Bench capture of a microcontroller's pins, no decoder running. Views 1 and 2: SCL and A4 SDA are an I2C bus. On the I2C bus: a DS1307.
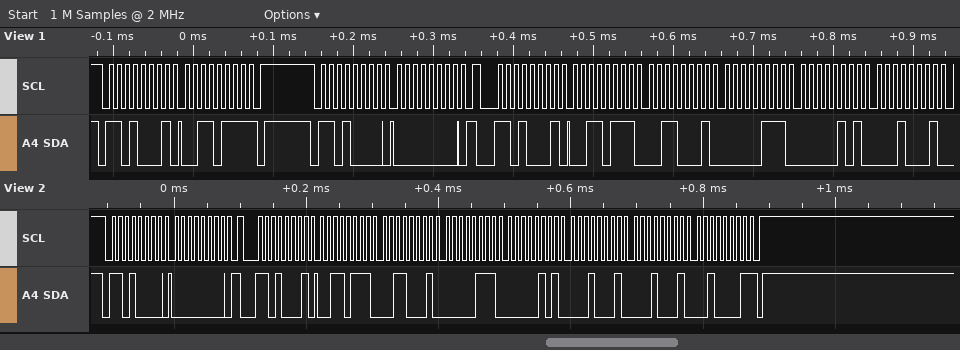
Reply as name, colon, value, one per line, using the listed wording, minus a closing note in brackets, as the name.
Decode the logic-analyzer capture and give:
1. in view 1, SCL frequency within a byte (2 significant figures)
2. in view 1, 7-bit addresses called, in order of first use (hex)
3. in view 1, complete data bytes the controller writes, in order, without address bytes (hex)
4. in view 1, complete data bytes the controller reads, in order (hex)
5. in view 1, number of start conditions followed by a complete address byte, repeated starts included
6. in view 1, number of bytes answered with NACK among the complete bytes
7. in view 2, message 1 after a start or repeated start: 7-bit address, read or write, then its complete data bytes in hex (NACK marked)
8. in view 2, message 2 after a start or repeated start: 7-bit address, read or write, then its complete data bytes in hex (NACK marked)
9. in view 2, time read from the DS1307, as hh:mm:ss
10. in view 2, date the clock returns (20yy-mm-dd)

in view 1, SCL frequency within a byte: 100 kHz
in view 1, 7-bit addresses called, in order of first use: 0x68
in view 1, complete data bytes the controller writes, in order, without address bytes: 00
in view 1, complete data bytes the controller reads, in order: 37 37 31 07 05 11
in view 1, number of start conditions followed by a complete address byte, repeated starts included: 3
in view 1, number of bytes answered with NACK among the complete bytes: 1
in view 2, message 1 after a start or repeated start: 7-bit address, read or write, then its complete data bytes in hex: 0x68 write: 00
in view 2, message 2 after a start or repeated start: 7-bit address, read or write, then its complete data bytes in hex: 0x68 read: 37 31 07 05 11 11 21 NACK
in view 2, time read from the DS1307, as hh:mm:ss: 07:31:37
in view 2, date the clock returns: 2021-11-11
